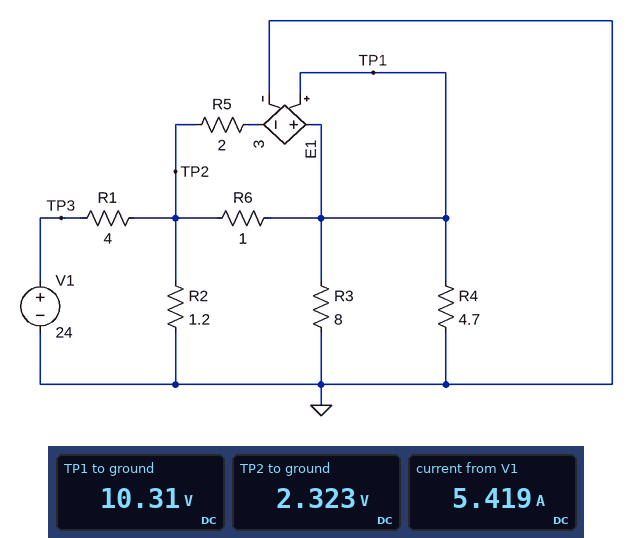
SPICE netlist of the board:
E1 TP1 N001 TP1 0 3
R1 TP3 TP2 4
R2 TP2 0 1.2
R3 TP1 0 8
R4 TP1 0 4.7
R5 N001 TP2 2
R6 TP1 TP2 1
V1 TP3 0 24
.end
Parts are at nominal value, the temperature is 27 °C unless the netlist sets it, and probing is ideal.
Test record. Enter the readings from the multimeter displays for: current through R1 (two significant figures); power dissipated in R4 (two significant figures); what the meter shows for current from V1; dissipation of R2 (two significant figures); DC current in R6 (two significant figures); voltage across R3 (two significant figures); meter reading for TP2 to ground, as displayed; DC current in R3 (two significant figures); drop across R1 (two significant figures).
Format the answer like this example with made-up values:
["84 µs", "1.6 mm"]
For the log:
["5.4 A", "23 W", "5.419 A", "4.5 W", "8.0 A", "10 V", "2.323 V", "1.3 A", "22 V"]
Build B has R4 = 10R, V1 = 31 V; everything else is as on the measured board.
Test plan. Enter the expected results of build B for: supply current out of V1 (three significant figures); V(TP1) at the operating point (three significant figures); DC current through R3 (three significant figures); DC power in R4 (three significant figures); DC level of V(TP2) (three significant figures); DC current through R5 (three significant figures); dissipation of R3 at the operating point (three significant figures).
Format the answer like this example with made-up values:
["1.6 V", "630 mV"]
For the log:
["7.00 A", "20.0 V", "2.50 A", "40.0 W", "3.00 V", "21.5 A", "50.0 W"]
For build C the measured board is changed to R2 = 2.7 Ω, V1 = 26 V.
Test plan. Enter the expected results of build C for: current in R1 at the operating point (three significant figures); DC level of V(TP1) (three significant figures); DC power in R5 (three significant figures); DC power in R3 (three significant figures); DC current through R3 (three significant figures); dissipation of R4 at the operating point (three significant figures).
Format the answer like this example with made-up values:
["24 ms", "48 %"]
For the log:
["5.73 A", "13.6 V", "459 W", "23.2 W", "1.70 A", "39.4 W"]
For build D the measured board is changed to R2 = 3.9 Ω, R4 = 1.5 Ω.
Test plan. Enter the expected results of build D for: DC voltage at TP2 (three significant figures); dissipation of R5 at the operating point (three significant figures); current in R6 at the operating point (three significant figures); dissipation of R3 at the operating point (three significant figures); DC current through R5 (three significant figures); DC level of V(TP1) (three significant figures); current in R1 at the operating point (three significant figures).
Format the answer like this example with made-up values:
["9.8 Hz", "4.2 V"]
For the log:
["2.99 V", "103 W", "2.68 A", "4.01 W", "7.16 A", "5.67 V", "5.25 A"]
